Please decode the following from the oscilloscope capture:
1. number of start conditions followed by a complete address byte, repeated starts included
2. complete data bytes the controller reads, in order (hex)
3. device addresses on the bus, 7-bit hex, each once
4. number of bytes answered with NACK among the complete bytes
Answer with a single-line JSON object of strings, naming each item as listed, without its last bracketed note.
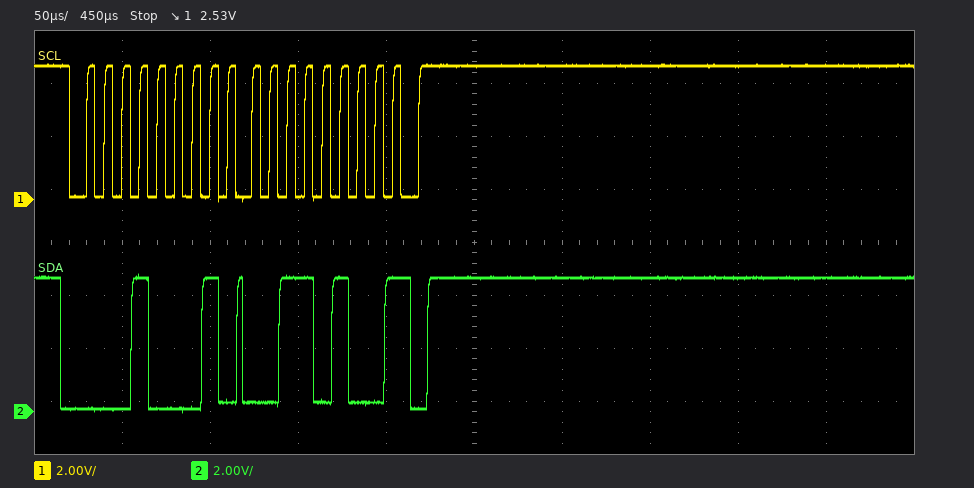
{"number of start conditions followed by a complete address byte, repeated starts included": "1", "complete data bytes the controller reads, in order": "34", "device addresses on the bus, 7-bit hex, each once": "0x08", "number of bytes answered with NACK among the complete bytes": "1"}
